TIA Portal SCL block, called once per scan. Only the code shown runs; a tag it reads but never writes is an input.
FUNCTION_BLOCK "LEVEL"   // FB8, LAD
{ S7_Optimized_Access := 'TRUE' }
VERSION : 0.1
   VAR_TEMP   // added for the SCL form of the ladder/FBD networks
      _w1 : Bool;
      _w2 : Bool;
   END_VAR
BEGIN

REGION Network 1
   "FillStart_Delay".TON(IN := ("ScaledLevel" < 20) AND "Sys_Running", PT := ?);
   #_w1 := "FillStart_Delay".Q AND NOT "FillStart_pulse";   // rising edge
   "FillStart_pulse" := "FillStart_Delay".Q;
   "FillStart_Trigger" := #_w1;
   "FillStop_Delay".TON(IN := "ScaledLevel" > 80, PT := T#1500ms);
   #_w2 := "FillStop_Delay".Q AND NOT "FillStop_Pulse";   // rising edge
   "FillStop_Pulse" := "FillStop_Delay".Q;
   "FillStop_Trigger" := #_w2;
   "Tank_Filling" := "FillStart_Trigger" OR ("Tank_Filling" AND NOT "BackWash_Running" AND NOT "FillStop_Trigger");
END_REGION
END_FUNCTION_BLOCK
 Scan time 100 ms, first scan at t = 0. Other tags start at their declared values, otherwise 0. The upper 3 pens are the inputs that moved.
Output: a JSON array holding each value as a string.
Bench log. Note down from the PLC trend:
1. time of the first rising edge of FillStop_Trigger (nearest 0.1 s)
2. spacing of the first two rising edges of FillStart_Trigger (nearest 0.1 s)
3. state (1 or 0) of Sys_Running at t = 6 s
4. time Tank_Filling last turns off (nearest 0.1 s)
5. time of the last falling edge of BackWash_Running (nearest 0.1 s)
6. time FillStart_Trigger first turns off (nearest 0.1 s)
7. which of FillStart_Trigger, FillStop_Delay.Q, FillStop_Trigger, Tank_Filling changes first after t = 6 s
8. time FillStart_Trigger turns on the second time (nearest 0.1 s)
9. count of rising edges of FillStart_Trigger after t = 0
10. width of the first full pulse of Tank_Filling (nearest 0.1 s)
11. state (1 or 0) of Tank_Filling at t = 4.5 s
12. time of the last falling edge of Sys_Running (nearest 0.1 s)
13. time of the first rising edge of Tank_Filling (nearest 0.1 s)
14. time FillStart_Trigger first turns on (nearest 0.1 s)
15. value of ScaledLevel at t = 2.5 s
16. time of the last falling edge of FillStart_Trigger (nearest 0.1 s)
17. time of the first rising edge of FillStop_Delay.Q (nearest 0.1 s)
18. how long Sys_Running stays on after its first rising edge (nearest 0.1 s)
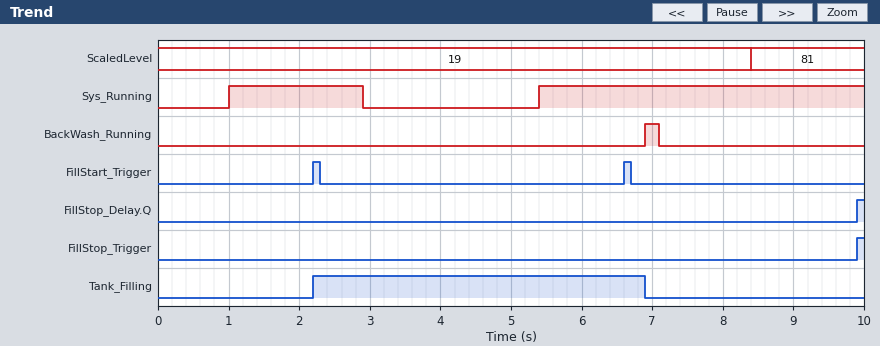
["9.9 s", "4.4 s", "1", "6.9 s", "7.1 s", "2.3 s", "FillStart_Trigger", "6.6 s", "2", "4.7 s", "1", "2.9 s", "2.2 s", "2.2 s", "19", "6.7 s", "9.9 s", "1.9 s"]
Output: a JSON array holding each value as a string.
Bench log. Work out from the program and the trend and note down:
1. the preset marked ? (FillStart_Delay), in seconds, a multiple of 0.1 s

["1.2 s"]
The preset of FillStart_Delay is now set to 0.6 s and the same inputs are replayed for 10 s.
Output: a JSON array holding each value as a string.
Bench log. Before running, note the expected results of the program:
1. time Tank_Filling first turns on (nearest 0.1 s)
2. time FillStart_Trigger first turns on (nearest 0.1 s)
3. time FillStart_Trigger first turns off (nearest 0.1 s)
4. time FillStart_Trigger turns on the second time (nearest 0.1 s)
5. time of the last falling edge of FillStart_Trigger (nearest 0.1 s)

["1.6 s", "1.6 s", "1.7 s", "6.0 s", "6.1 s"]
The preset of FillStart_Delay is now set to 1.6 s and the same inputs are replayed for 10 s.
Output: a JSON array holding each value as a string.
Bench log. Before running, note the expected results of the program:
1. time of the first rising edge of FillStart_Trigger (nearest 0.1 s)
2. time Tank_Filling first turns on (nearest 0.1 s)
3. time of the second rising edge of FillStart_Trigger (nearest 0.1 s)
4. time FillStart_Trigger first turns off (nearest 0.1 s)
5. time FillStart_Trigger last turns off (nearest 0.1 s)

["2.6 s", "2.6 s", "7.0 s", "2.7 s", "7.1 s"]
